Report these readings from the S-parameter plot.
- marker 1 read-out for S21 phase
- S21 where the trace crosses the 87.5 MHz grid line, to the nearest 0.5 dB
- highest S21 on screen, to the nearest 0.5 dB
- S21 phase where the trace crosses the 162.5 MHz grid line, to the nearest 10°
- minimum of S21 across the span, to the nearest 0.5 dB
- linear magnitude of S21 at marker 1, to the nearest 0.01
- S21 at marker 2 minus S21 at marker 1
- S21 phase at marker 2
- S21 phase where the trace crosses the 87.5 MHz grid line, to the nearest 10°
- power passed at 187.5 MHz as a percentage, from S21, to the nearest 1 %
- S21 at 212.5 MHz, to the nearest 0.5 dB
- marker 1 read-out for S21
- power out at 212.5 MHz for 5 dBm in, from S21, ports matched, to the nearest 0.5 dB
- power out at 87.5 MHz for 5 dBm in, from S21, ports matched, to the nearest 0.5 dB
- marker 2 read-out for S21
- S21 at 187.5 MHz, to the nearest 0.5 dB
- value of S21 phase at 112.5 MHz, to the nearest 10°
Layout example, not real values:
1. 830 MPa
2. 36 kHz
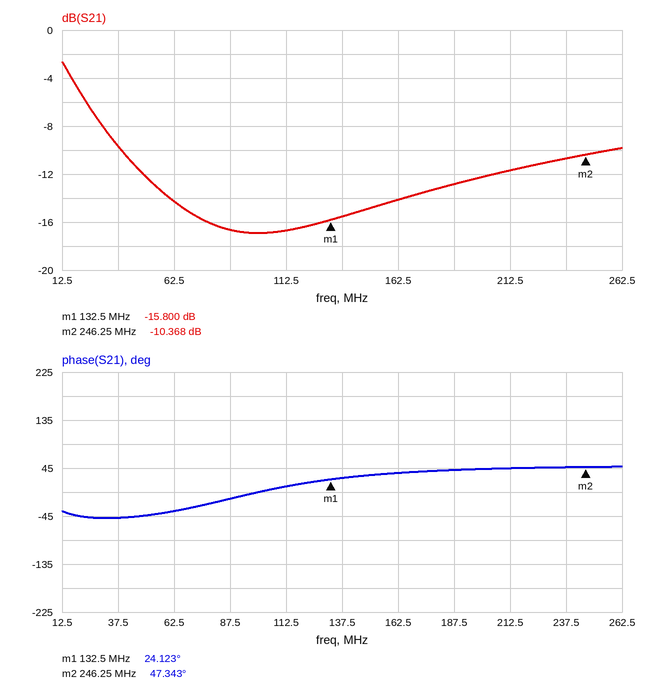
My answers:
1. 24.123°
2. -16.5 dB
3. -2.5 dB
4. 40°
5. -17.0 dB
6. 0.16
7. 5.432 dB
8. 47.343°
9. -10°
10. 5 %
11. -11.5 dB
12. -15.800 dB
13. -6.5 dBm
14. -11.5 dBm
15. -10.368 dB
16. -13.0 dB
17. 10°
